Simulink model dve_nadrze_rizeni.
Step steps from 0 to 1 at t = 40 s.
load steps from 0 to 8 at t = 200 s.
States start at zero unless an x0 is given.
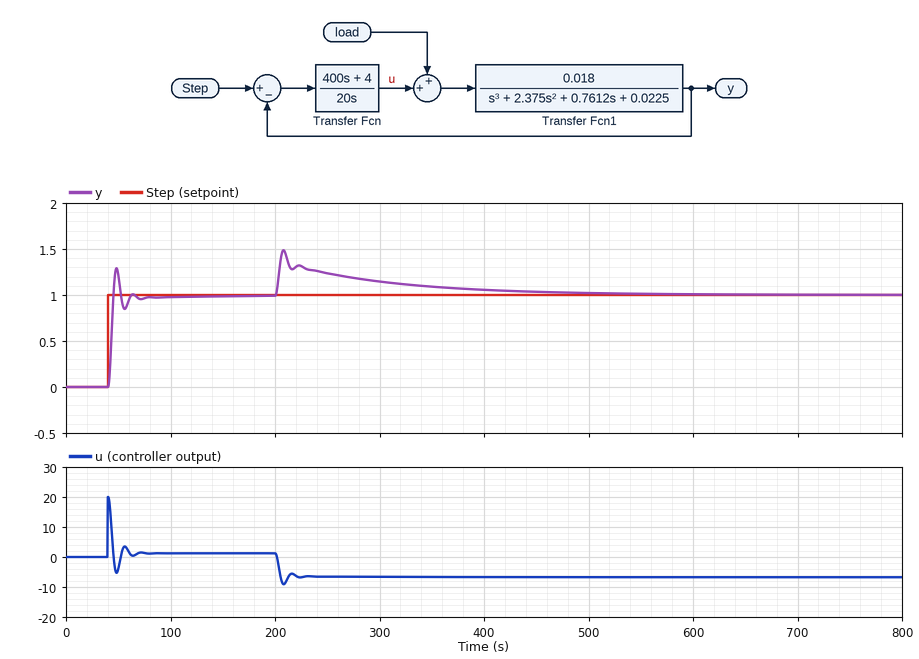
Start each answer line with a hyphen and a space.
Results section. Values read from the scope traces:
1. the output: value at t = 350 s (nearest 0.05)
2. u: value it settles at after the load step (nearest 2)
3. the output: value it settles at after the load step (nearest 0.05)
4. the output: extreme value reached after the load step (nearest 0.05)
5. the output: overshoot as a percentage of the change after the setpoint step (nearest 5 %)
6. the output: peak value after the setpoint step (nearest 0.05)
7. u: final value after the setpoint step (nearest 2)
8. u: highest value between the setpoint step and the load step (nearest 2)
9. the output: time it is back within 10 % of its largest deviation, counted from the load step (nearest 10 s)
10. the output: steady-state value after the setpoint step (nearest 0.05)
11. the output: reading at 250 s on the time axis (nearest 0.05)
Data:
- 1.10
- -6
- 1.00
- 1.50
- 30 %
- 1.30
- 2
- 20
- 210 s
- 1.00
- 1.25
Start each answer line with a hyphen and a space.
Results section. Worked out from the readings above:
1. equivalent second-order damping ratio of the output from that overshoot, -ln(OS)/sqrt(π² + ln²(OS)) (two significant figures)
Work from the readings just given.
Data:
- 0.36
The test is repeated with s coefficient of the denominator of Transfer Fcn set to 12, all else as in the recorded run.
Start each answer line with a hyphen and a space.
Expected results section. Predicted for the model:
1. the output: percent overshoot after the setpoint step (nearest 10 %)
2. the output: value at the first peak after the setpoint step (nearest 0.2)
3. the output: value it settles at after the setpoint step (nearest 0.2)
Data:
- 50 %
- 1.4
- 1.0
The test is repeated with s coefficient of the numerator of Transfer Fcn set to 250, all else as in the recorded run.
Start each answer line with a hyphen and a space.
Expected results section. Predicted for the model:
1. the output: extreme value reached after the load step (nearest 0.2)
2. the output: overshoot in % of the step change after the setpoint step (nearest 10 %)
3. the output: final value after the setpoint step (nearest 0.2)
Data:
- 1.6
- 20 %
- 1.0
